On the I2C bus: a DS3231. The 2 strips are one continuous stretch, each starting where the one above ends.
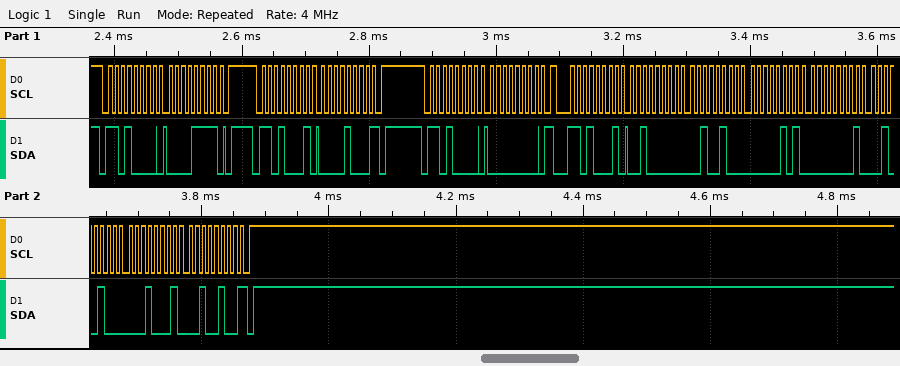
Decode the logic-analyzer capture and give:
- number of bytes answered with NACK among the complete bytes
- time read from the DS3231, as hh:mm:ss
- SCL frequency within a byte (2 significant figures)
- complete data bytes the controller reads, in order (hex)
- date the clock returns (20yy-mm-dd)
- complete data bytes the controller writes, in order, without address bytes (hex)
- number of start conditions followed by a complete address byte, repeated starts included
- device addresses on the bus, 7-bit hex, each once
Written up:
2
05:24:20
100 kHz
08 20 24 05 01 24 11 24
2024-11-24
0F 00
4
0x68
